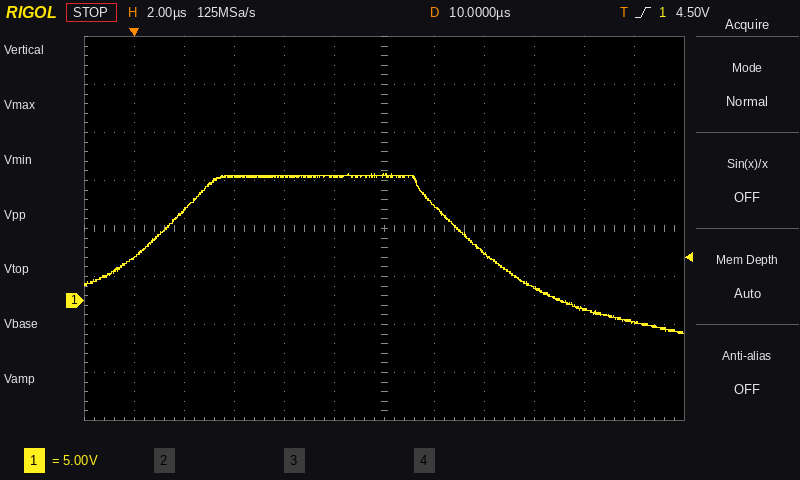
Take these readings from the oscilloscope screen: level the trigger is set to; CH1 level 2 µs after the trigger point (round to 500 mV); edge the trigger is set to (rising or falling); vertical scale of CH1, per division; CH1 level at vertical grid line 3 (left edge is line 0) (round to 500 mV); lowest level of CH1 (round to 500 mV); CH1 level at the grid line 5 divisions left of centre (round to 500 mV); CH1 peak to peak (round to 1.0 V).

4.50 V
9.5 V
rising
5 V
13.0 V
-3.5 V
4.5 V
17.0 V
